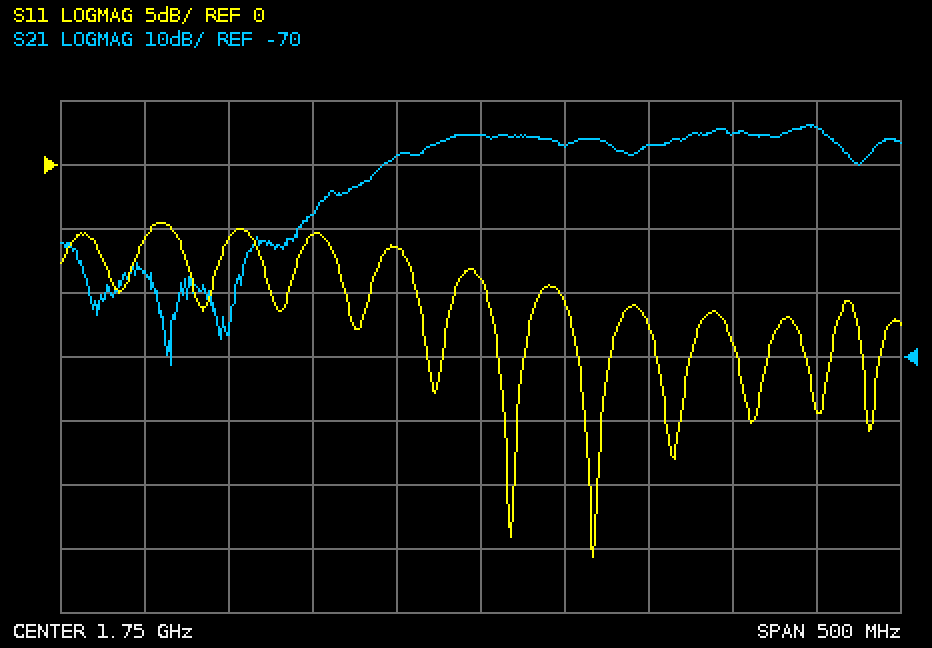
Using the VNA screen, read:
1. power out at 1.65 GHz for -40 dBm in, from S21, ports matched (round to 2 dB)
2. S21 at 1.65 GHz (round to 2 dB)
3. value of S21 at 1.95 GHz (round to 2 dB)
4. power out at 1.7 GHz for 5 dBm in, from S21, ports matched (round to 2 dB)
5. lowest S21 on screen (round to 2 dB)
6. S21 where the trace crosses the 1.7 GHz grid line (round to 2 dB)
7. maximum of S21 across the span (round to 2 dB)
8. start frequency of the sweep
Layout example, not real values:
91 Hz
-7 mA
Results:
-88 dBm
-48 dB
-34 dB
-34 dBm
-72 dB
-38 dB
-34 dB
1.5 GHz
